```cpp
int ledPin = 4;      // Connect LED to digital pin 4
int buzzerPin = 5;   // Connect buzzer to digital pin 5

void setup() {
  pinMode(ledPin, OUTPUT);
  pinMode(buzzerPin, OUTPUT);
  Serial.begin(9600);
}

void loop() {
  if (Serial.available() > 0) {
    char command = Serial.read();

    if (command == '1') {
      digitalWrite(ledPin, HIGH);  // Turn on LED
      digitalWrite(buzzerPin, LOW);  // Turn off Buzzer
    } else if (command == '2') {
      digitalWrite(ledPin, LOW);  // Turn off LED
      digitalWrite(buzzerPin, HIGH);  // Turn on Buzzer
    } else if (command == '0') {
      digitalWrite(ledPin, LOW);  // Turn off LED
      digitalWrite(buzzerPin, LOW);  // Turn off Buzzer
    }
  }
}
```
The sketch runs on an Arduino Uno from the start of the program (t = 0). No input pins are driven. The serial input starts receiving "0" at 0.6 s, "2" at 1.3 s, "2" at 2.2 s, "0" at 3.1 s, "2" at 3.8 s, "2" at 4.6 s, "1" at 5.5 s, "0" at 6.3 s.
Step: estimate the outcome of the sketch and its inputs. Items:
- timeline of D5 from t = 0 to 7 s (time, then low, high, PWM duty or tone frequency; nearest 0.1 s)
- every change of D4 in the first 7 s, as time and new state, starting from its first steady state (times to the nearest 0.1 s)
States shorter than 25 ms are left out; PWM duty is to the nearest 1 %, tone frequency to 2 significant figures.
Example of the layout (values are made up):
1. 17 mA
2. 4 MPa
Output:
1. 0 s low; 1.3 s high; 3.1 s low; 3.8 s high; 5.5 s low
2. 0 s low; 5.5 s high; 6.3 s low
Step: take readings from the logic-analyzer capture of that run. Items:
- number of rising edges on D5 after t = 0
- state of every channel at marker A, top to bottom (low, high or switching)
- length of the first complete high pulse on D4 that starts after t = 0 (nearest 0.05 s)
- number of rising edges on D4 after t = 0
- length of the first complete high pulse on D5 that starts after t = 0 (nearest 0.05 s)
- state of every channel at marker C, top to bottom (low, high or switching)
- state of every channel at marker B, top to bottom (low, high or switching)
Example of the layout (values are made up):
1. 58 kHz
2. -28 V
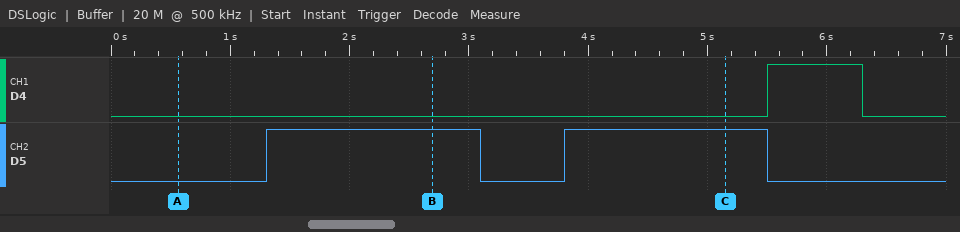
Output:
1. 2
2. D4 low, D5 low
3. 0.80 s
4. 1
5. 1.80 s
6. D4 low, D5 high
7. D4 low, D5 high
